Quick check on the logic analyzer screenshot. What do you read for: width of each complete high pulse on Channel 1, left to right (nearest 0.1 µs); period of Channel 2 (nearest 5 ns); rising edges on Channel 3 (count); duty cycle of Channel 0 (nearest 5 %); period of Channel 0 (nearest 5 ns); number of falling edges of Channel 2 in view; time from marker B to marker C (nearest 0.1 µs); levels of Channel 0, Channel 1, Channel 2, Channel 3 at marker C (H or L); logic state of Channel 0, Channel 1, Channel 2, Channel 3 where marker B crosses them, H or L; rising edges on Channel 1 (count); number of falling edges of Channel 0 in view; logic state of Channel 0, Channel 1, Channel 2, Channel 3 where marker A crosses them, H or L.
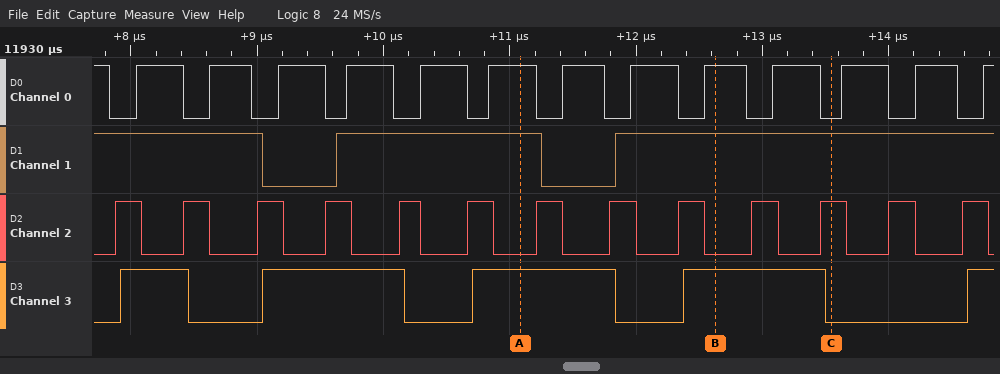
1.6 µs
560 ns
5
65 %
560 ns
13
0.9 µs
Channel 0=L, Channel 1=H, Channel 2=H, Channel 3=L
Channel 0=H, Channel 1=H, Channel 2=L, Channel 3=H
2
13
Channel 0=H, Channel 1=H, Channel 2=L, Channel 3=H
